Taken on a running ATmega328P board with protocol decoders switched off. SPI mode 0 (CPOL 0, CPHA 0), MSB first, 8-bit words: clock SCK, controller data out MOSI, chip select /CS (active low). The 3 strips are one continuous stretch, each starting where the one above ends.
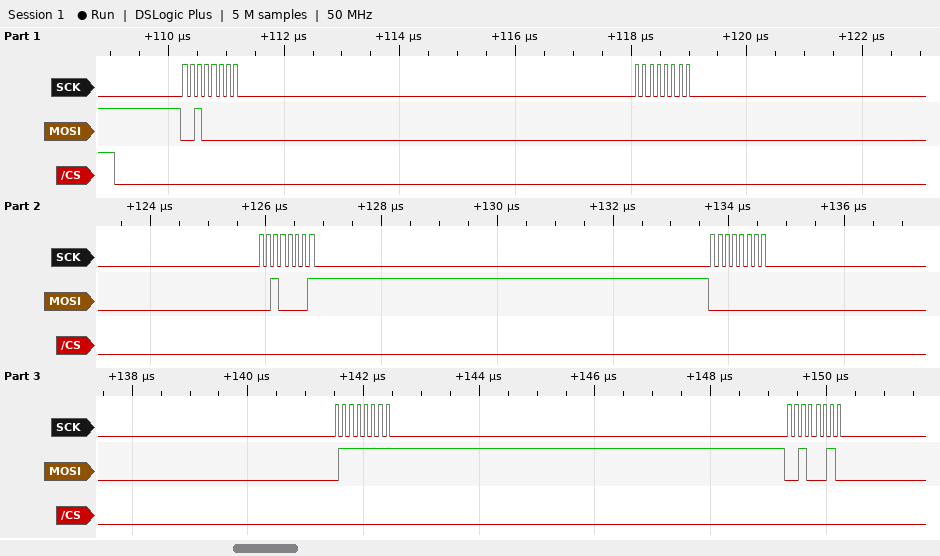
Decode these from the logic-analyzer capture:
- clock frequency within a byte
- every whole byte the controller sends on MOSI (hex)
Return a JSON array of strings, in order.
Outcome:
["8 MHz", "20 00 21 00 7F 22"]
